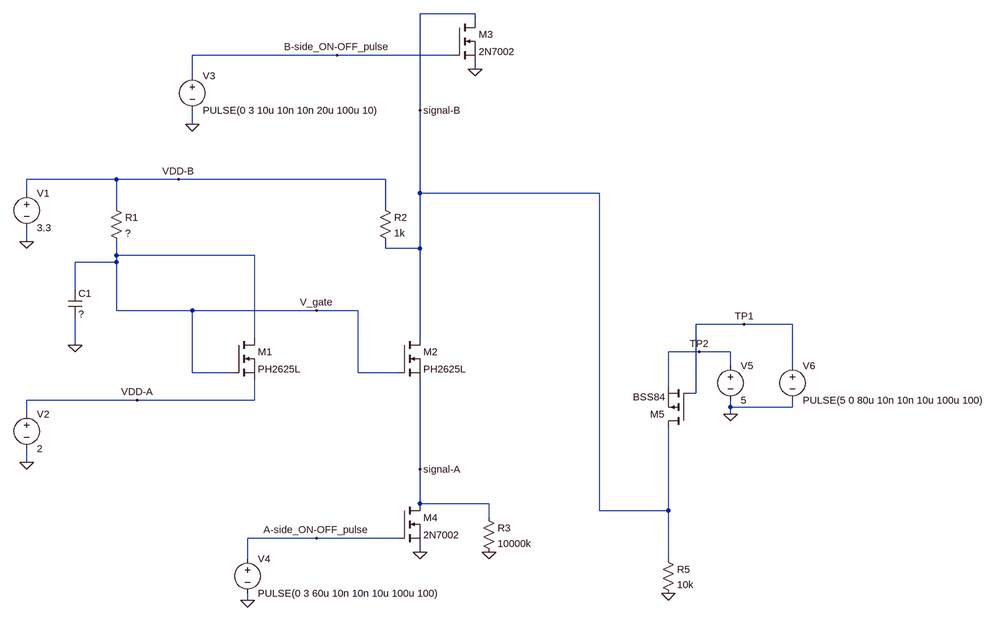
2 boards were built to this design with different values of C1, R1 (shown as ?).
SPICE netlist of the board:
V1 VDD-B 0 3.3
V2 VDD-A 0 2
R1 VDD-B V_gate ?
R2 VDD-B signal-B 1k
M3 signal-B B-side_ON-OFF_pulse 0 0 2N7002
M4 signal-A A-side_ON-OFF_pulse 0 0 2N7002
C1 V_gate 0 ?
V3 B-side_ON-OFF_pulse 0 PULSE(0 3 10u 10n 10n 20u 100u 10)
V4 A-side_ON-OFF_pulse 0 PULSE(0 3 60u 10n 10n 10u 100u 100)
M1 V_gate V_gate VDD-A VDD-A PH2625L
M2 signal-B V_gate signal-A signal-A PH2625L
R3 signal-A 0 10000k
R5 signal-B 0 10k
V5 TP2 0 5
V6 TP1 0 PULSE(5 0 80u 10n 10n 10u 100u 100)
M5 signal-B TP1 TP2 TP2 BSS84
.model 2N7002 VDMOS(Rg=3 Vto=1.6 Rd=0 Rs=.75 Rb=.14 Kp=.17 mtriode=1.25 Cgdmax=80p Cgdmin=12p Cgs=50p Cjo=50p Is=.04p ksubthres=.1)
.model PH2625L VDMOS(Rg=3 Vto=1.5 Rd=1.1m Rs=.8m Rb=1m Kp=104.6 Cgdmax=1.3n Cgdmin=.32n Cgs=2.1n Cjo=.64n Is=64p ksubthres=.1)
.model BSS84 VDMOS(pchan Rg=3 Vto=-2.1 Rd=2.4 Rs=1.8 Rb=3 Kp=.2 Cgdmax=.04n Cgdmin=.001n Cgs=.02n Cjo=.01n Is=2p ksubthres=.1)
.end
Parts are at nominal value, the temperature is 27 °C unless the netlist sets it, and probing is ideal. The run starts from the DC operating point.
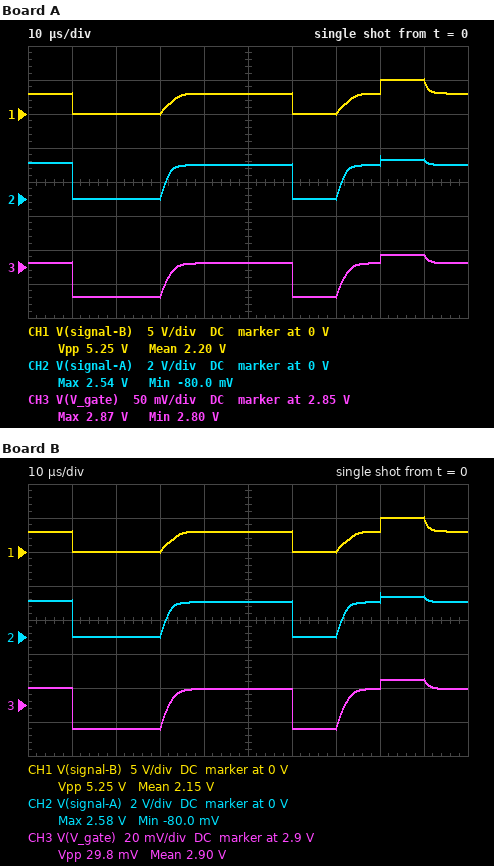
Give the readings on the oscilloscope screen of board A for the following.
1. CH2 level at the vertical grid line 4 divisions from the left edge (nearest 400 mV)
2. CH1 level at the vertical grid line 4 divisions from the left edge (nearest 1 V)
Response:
2.0 V
3 V
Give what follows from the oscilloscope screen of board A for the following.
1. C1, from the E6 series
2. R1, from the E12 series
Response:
150 nF
330 kΩ
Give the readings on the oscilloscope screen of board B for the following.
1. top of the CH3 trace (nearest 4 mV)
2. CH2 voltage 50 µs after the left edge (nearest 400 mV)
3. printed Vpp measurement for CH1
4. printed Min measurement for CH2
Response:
2.916 V
2.0 V
5.25 V
-80.0 mV
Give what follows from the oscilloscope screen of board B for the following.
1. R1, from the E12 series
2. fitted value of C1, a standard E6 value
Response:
100 kΩ
330 nF
